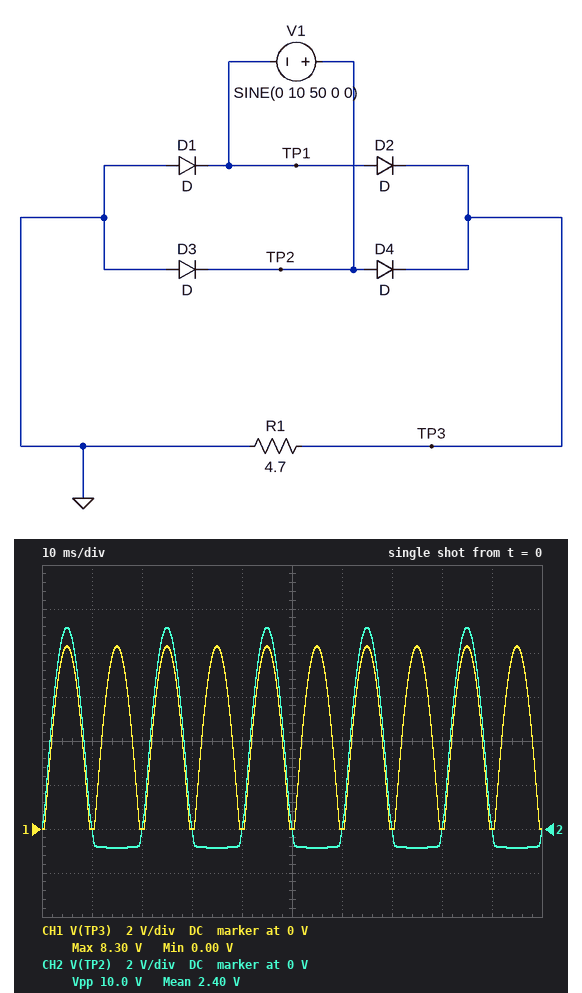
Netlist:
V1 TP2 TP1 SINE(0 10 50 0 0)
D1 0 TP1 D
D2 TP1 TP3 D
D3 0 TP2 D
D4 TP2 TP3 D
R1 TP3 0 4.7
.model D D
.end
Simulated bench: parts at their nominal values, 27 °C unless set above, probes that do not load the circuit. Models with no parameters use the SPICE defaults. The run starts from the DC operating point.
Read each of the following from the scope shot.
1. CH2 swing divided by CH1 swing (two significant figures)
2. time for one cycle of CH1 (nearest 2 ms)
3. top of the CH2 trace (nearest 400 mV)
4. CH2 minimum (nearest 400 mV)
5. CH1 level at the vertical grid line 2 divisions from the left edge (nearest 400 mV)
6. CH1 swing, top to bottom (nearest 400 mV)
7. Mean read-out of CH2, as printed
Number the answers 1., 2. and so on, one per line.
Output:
1. 1.2
2. 10 ms
3. 9.2 V
4. -800 mV
5. 0 V
6. 8.4 V
7. 2.40 V
